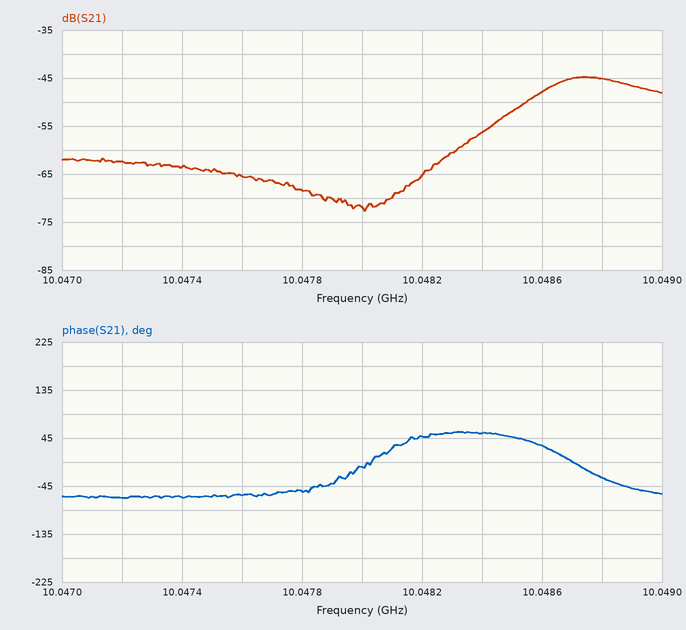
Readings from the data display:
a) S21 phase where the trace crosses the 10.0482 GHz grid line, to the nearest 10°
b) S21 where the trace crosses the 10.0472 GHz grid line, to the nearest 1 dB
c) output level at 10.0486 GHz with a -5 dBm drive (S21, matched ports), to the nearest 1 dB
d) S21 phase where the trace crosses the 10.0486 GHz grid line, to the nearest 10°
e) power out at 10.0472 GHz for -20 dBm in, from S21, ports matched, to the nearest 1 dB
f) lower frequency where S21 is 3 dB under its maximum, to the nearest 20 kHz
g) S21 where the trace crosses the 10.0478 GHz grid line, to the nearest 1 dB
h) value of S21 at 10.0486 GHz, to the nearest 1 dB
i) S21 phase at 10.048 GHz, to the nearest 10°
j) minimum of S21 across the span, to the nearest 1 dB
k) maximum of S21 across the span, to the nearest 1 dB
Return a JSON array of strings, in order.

["50°", "-62 dB", "-53 dBm", "30°", "-82 dBm", "10.04860 GHz", "-68 dB", "-48 dB", "-10°", "-73 dB", "-45 dB"]
